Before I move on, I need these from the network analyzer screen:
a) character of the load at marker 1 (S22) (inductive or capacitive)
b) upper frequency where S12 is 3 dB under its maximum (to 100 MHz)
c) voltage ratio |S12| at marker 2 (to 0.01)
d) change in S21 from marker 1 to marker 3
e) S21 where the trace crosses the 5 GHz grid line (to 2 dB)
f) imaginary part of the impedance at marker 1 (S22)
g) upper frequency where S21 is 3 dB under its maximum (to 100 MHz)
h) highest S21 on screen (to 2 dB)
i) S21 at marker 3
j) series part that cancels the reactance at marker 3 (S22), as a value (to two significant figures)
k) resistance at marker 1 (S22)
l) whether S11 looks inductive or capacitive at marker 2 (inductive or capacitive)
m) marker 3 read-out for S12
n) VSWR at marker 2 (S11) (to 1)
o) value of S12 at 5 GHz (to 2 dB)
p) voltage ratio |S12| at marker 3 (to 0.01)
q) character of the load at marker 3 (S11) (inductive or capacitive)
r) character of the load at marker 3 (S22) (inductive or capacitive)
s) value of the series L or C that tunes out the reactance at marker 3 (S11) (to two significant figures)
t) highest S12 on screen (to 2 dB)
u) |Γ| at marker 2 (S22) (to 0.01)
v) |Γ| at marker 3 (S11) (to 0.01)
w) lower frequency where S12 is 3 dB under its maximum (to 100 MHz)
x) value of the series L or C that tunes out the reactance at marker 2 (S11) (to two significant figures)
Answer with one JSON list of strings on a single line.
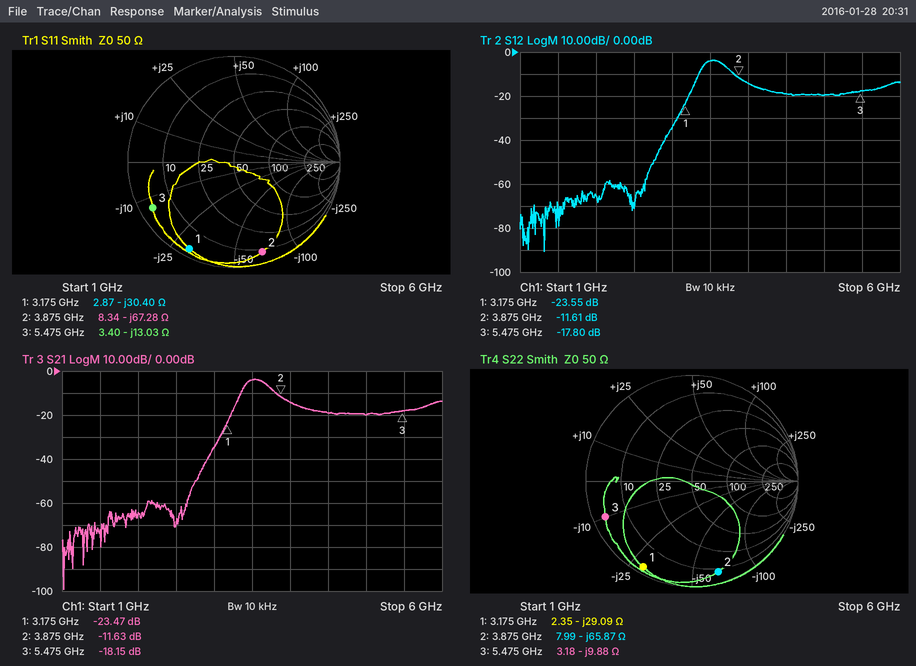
["capacitive", "3.7 GHz", "0.26", "5.32 dB", "-20 dB", "-29.09 Ω", "3.7 GHz", "-4 dB", "-18.15 dB", "290 pH", "2.35 Ω", "capacitive", "-17.80 dB", "17", "-20 dB", "0.13", "capacitive", "capacitive", "380 pH", "-4 dB", "0.89", "0.88", "3.4 GHz", "2.8 nH"]
